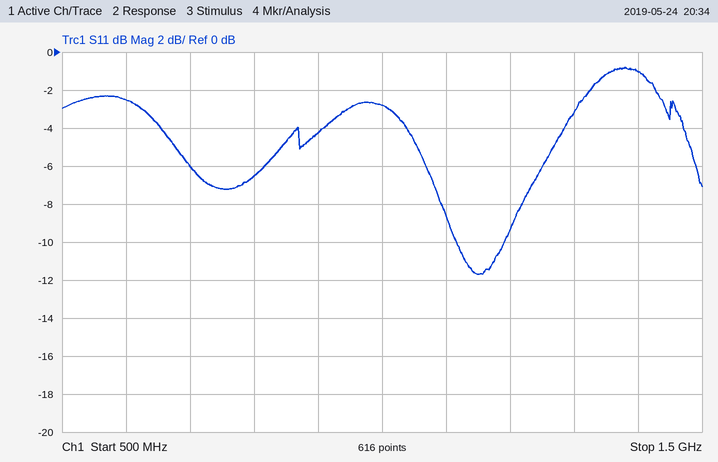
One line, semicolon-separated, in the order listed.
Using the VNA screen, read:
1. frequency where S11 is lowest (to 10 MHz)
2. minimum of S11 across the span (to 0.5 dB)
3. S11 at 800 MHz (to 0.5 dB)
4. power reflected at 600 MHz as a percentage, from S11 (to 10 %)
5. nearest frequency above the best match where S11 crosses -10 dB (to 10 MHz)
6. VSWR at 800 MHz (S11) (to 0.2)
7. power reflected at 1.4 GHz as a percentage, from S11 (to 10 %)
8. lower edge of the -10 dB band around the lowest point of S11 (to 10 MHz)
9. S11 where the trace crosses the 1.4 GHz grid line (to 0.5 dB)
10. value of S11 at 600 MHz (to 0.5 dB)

1.15 GHz; -11.5 dB; -6.5 dB; 60 %; 1.19 GHz; 2.8; 80 %; 1.12 GHz; -1.0 dB; -2.5 dB
